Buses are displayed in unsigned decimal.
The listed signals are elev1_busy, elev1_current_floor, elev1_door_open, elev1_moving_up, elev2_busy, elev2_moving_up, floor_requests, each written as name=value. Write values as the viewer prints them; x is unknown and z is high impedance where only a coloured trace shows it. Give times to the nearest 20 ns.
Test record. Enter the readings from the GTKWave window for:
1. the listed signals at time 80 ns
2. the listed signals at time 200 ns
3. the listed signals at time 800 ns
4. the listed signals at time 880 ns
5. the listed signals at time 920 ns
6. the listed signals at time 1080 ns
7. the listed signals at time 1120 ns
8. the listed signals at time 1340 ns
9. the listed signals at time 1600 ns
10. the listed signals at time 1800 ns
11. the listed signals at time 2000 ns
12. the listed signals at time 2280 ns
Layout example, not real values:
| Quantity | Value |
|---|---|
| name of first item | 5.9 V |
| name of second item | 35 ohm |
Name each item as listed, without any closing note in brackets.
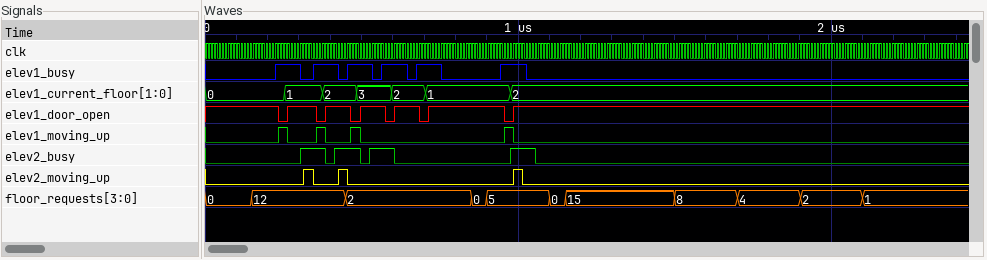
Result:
| Quantity | Value |
|---|---|
| the listed signals at time 80 ns | elev1_busy=0, elev1_current_floor=0, elev1_door_open=1, elev1_moving_up=0, elev2_busy=0, elev2_moving_up=0, floor_requests=0 |
| the listed signals at time 200 ns | elev1_busy=0, elev1_current_floor=0, elev1_door_open=1, elev1_moving_up=0, elev2_busy=0, elev2_moving_up=0, floor_requests=12 |
| the listed signals at time 800 ns | elev1_busy=0, elev1_current_floor=1, elev1_door_open=1, elev1_moving_up=0, elev2_busy=0, elev2_moving_up=0, floor_requests=2 |
| the listed signals at time 880 ns | elev1_busy=0, elev1_current_floor=1, elev1_door_open=1, elev1_moving_up=0, elev2_busy=0, elev2_moving_up=0, floor_requests=0 |
| the listed signals at time 920 ns | elev1_busy=0, elev1_current_floor=1, elev1_door_open=1, elev1_moving_up=0, elev2_busy=0, elev2_moving_up=0, floor_requests=5 |
| the listed signals at time 1080 ns | elev1_busy=0, elev1_current_floor=2, elev1_door_open=1, elev1_moving_up=0, elev2_busy=0, elev2_moving_up=0, floor_requests=5 |
| the listed signals at time 1120 ns | elev1_busy=0, elev1_current_floor=2, elev1_door_open=1, elev1_moving_up=0, elev2_busy=0, elev2_moving_up=0, floor_requests=0 |
| the listed signals at time 1340 ns | elev1_busy=0, elev1_current_floor=2, elev1_door_open=1, elev1_moving_up=0, elev2_busy=0, elev2_moving_up=0, floor_requests=15 |
| the listed signals at time 1600 ns | elev1_busy=0, elev1_current_floor=2, elev1_door_open=1, elev1_moving_up=0, elev2_busy=0, elev2_moving_up=0, floor_requests=8 |
| the listed signals at time 1800 ns | elev1_busy=0, elev1_current_floor=2, elev1_door_open=1, elev1_moving_up=0, elev2_busy=0, elev2_moving_up=0, floor_requests=4 |
| the listed signals at time 2000 ns | elev1_busy=0, elev1_current_floor=2, elev1_door_open=1, elev1_moving_up=0, elev2_busy=0, elev2_moving_up=0, floor_requests=2 |
| the listed signals at time 2280 ns | elev1_busy=0, elev1_current_floor=2, elev1_door_open=1, elev1_moving_up=0, elev2_busy=0, elev2_moving_up=0, floor_requests=1 |
